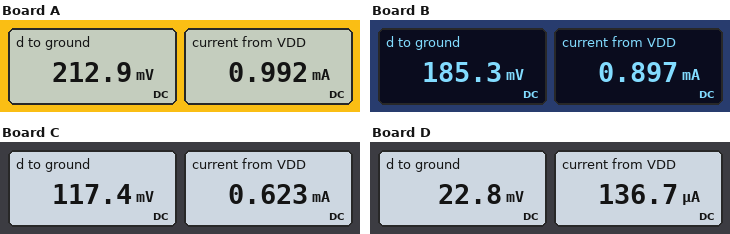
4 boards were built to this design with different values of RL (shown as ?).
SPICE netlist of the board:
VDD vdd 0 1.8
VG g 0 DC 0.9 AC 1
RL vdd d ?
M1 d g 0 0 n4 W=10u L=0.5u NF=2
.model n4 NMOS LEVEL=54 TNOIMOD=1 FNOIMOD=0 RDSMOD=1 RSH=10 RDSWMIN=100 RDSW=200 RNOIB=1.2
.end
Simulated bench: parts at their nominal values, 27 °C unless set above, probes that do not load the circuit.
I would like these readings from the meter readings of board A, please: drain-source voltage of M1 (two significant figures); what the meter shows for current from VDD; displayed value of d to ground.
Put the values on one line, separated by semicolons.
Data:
210 mV; 0.992 mA; 212.9 mV
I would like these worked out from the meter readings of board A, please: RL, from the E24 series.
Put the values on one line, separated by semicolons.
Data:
1.6 kΩ
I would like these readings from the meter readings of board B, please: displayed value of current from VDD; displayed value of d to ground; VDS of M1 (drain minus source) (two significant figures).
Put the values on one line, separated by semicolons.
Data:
0.897 mA; 185.3 mV; 190 mV
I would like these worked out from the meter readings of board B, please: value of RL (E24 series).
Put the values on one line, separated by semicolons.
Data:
1.8 kΩ
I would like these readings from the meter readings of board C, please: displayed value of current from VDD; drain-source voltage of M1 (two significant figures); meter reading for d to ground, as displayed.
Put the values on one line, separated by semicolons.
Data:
0.623 mA; 120 mV; 117.4 mV
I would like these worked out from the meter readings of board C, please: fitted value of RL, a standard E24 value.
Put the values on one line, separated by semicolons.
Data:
2.7 kΩ
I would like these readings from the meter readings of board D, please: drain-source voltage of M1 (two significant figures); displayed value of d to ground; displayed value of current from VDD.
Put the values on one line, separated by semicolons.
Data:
23 mV; 22.8 mV; 136.7 µA
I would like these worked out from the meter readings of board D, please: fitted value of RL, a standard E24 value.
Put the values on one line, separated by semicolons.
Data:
13 kΩ
